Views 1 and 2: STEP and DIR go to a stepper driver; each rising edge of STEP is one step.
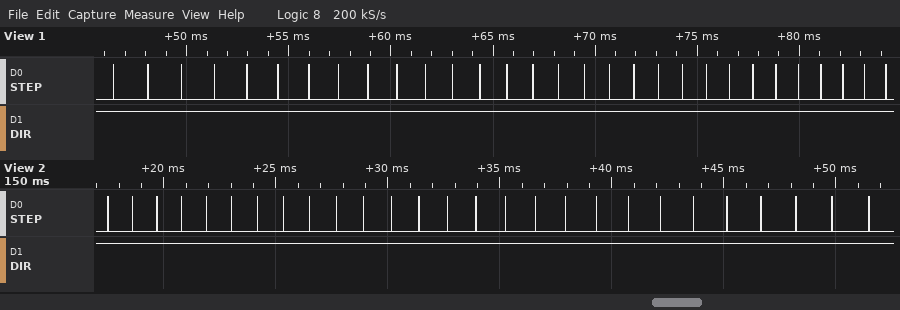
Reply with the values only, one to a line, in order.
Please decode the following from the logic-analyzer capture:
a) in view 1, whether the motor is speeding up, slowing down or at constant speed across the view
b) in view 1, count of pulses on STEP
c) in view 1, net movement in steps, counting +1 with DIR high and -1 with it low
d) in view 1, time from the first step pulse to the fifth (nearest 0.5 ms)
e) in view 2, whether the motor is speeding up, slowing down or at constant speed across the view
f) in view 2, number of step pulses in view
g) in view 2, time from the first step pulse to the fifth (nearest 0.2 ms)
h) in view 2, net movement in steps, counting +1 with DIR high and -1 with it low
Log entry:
speeding up
30
+30
6.5 ms
slowing down
27
4.4 ms
+27
